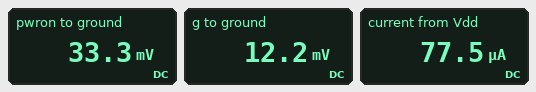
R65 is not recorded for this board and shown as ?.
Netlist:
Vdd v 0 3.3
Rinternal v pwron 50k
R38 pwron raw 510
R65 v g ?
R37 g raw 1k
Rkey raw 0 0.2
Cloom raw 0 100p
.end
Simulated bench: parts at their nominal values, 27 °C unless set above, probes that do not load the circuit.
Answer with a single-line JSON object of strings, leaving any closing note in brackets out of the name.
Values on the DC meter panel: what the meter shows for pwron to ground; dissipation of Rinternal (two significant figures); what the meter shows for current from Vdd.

{"what the meter shows for pwron to ground": "33.3 mV", "dissipation of Rinternal": "210 µW", "what the meter shows for current from Vdd": "77.5 µA"}
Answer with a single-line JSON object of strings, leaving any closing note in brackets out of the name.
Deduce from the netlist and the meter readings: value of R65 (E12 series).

{"value of R65": "270 kΩ"}
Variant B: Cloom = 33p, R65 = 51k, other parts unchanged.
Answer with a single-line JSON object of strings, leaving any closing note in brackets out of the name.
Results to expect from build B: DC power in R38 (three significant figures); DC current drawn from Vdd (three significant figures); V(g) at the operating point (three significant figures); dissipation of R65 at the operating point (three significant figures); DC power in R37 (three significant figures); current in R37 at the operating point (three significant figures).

{"DC power in R38": "2.18 µW", "DC current drawn from Vdd": "129 µA", "V(g) at the operating point": "63.5 mV", "dissipation of R65 at the operating point": "205 µW", "DC power in R37": "4.03 µW", "current in R37 at the operating point": "63.5 µA"}
